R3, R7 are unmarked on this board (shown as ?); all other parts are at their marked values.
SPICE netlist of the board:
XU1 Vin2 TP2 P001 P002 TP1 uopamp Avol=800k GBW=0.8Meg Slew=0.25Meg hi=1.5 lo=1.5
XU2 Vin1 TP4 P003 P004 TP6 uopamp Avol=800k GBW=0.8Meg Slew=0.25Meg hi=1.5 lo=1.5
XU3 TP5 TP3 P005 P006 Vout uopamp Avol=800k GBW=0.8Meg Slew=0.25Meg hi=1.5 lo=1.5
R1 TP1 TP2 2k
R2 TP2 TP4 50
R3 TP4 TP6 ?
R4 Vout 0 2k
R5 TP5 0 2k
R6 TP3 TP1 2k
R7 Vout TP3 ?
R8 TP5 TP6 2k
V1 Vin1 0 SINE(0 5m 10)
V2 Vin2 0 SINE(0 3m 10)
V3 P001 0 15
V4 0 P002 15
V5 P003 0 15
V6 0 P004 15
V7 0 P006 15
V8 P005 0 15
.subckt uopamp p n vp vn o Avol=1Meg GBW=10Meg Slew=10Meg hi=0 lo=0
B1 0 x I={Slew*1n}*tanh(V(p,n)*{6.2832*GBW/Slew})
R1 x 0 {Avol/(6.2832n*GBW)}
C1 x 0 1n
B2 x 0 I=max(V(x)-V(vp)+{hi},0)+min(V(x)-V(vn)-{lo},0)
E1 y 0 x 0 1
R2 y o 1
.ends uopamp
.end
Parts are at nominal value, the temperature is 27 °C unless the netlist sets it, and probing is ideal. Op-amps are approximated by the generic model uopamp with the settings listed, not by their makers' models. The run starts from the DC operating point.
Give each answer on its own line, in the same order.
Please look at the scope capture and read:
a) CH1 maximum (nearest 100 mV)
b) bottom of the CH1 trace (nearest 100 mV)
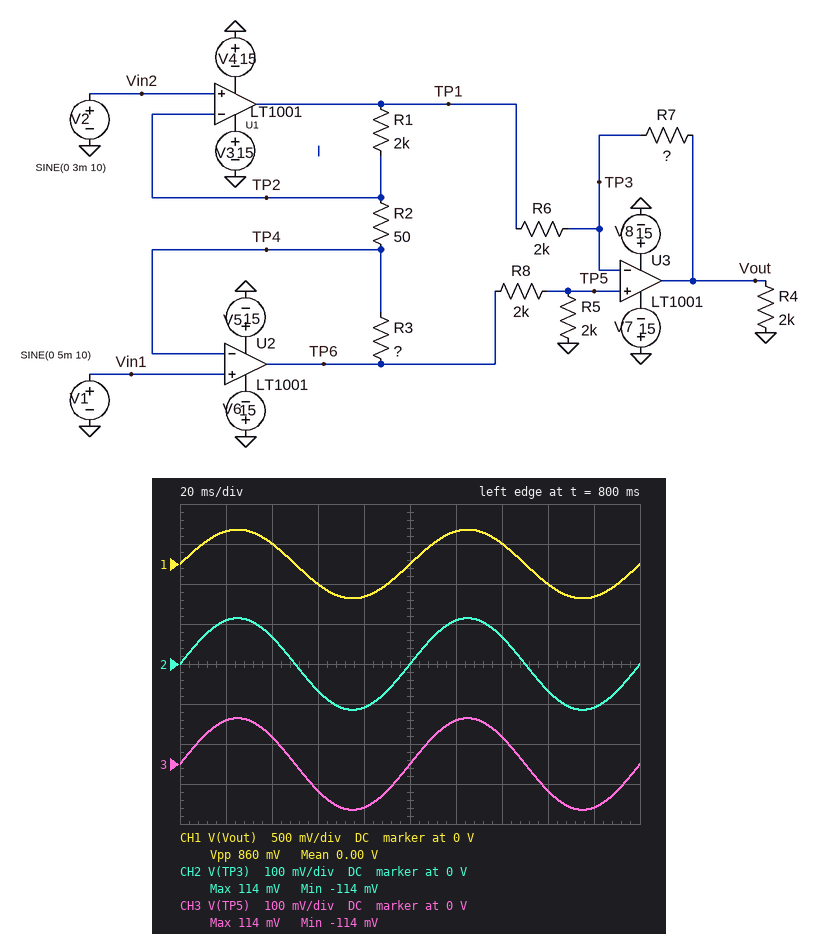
400 mV
-400 mV
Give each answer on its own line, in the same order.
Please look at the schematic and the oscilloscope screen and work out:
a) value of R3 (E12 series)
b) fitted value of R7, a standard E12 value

5.6 kΩ
3.3 kΩ
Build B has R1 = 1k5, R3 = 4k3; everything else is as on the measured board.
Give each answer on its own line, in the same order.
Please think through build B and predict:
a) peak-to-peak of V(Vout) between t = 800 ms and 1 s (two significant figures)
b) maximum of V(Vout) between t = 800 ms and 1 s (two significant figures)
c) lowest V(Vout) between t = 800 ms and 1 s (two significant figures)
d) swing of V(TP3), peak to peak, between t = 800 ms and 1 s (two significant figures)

660 mV
330 mV
-330 mV
180 mV
